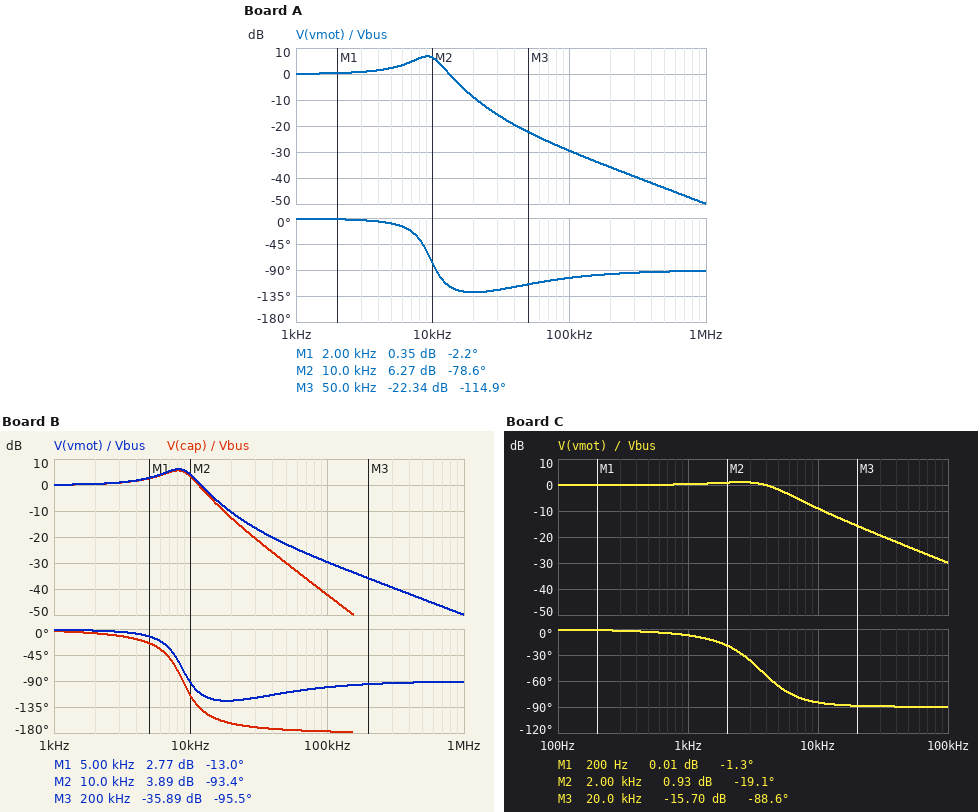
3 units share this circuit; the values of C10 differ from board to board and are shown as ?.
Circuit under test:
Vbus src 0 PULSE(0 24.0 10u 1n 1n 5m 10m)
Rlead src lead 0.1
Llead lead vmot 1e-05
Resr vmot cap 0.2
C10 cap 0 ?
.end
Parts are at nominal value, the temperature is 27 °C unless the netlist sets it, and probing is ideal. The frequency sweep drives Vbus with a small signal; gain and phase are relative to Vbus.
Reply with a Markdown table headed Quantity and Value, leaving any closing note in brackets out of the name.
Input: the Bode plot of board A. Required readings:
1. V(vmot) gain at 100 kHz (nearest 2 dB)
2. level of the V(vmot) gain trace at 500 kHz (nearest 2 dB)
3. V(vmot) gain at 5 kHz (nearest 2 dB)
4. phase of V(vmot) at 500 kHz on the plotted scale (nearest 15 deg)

| Quantity | Value |
|---|---|
| V(vmot) gain at 100 kHz | -30 dB |
| level of the V(vmot) gain trace at 500 kHz | -44 dB |
| V(vmot) gain at 5 kHz | 2 dB |
| phase of V(vmot) at 500 kHz on the plotted scale | -90 deg |
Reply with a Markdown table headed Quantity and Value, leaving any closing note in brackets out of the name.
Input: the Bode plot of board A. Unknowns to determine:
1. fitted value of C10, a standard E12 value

| Quantity | Value |
|---|---|
| fitted value of C10, a standard E12 value | 27 µF |
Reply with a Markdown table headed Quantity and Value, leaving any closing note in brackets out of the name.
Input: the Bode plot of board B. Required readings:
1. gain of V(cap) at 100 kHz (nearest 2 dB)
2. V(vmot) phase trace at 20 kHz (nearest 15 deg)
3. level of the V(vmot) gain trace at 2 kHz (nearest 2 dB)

| Quantity | Value |
|---|---|
| gain of V(cap) at 100 kHz | -42 dB |
| V(vmot) phase trace at 20 kHz | -120 deg |
| level of the V(vmot) gain trace at 2 kHz | 0 dB |
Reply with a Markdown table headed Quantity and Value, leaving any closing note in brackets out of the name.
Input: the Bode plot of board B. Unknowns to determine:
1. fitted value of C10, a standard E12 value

| Quantity | Value |
|---|---|
| fitted value of C10, a standard E12 value | 33 µF |
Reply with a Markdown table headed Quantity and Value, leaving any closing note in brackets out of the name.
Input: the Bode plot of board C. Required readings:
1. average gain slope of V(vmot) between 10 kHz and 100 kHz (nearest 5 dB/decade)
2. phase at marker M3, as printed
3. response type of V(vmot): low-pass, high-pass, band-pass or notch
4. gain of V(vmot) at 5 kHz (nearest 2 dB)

| Quantity | Value |
|---|---|
| average gain slope of V(vmot) between 10 kHz and 100 kHz | -20 dB/decade |
| phase at marker M3, as printed | -88.6 deg |
| response type of V(vmot): low-pass, high-pass, band-pass or notch | low-pass |
| gain of V(vmot) at 5 kHz | -2 dB |
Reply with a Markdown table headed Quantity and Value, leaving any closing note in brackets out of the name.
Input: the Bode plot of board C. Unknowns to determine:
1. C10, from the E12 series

| Quantity | Value |
|---|---|
| C10, from the E12 series | 180 µF |
